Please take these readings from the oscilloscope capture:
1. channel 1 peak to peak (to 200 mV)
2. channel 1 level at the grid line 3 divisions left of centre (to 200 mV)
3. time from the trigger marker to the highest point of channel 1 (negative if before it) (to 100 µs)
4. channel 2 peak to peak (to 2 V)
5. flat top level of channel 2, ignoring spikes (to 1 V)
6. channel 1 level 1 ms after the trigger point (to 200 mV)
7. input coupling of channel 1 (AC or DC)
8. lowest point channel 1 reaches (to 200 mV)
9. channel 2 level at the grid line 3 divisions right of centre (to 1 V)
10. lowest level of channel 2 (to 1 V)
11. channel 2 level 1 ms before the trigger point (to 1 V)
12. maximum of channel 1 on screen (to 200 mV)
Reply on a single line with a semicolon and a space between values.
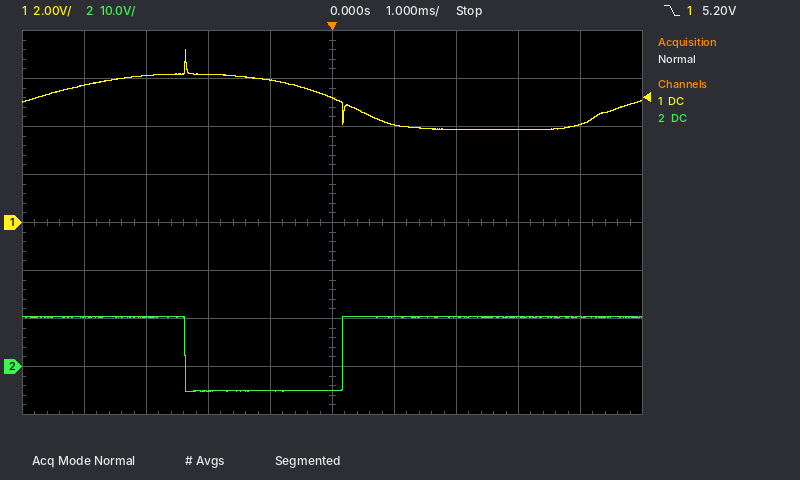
3.4 V; 6.2 V; -2.4 ms; 16 V; 10 V; 4.0 V; DC; 3.8 V; 10 V; -5 V; -5 V; 7.2 V
